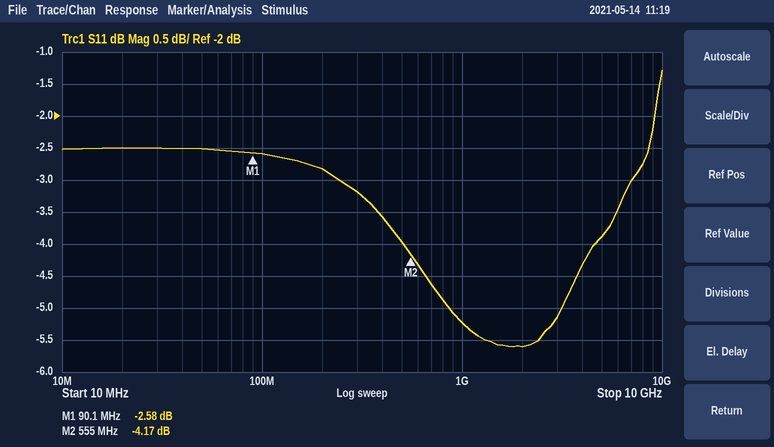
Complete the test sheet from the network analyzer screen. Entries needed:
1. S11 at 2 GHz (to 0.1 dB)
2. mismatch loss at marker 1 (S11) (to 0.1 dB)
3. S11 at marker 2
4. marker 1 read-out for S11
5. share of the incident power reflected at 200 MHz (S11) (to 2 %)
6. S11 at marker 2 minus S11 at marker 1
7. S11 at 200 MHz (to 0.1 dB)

-5.6 dB
3.5 dB
-4.17 dB
-2.58 dB
52 %
-1.59 dB
-2.8 dB
